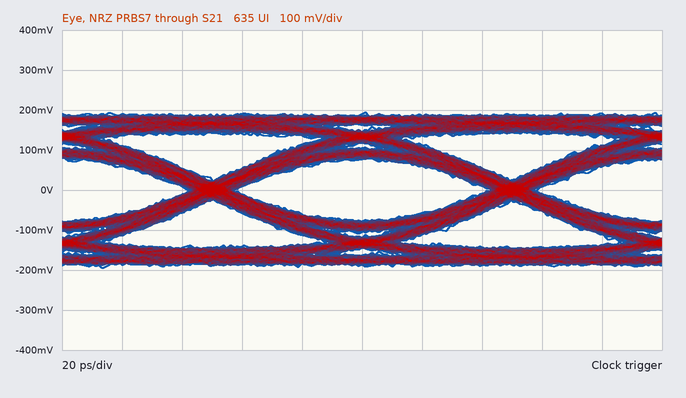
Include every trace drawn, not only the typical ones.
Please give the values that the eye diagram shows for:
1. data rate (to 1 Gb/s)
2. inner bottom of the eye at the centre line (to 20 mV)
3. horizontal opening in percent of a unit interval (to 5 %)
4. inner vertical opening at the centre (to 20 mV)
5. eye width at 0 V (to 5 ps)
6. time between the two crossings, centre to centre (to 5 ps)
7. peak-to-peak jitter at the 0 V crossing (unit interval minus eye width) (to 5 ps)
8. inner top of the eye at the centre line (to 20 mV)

10 Gb/s
-80 mV
85 %
160 mV
85 ps
100 ps
15 ps
80 mV
